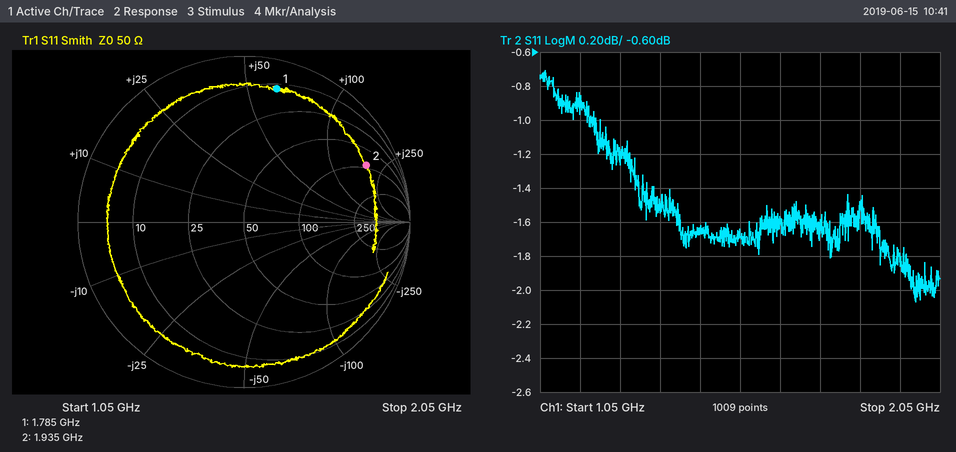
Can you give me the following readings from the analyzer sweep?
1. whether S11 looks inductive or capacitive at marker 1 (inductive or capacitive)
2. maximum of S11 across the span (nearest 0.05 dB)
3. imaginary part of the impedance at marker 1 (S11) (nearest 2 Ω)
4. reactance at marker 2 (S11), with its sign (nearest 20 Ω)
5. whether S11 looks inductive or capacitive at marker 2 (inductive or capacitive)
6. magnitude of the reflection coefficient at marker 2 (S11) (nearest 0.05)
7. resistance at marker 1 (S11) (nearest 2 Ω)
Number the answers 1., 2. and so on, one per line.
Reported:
1. inductive
2. -0.70 dB
3. +62 Ω
4. +180 Ω
5. inductive
6. 0.80
7. 12 Ω
